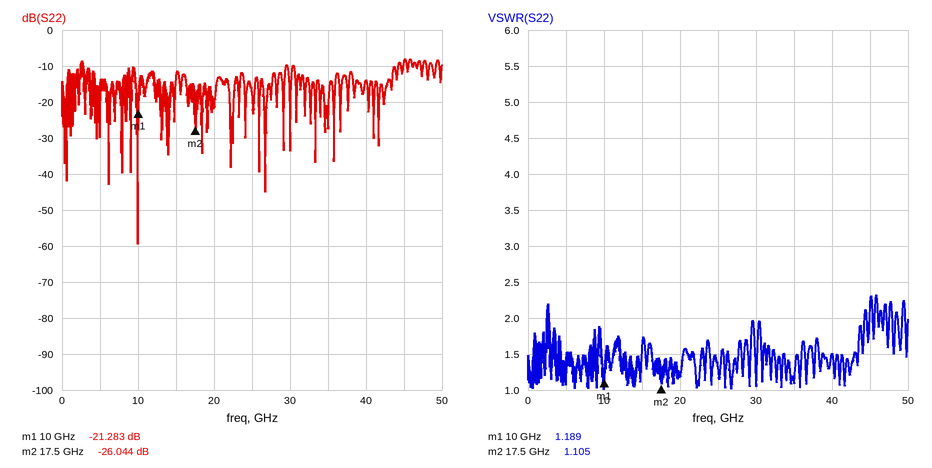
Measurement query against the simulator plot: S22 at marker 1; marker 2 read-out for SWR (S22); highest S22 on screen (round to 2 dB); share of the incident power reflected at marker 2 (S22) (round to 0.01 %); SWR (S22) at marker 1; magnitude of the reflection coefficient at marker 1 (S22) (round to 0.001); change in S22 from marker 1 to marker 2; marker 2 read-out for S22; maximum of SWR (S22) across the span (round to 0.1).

-21.283 dB
1.105
-8 dB
0.25 %
1.189
0.086
-4.761 dB
-26.044 dB
2.3
